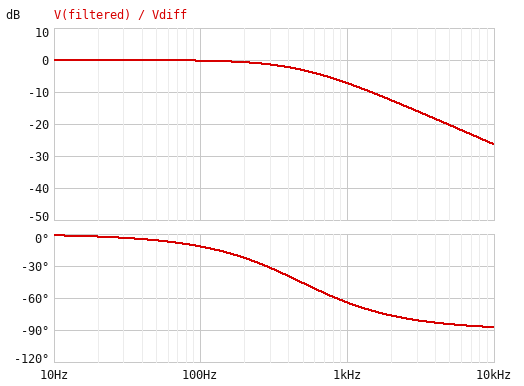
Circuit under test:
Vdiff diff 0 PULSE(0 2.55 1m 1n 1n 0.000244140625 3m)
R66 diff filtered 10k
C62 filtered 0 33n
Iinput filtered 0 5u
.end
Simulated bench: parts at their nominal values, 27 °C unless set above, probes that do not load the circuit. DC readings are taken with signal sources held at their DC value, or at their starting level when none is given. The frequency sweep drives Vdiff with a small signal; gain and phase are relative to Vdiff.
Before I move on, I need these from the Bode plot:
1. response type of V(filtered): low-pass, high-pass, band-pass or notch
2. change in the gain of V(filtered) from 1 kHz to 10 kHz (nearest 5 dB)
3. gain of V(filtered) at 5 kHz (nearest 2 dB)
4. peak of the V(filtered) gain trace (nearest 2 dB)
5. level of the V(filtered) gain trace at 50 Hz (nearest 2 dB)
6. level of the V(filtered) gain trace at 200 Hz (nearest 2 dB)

low-pass
-20 dB
-20 dB
0 dB
0 dB
0 dB
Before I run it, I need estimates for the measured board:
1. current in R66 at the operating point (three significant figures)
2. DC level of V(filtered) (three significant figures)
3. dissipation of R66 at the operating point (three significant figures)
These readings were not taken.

5.00 µA
-50.0 mV
250 nW
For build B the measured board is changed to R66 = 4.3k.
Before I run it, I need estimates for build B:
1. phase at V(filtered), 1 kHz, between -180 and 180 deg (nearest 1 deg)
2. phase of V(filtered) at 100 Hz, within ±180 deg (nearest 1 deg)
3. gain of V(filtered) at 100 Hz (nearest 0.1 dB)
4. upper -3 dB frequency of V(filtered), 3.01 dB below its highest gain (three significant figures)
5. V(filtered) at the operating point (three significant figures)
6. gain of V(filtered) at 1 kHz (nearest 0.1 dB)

-42 deg
-5 deg
0 dB
1.12 kHz
-21.5 mV
-2.5 dB
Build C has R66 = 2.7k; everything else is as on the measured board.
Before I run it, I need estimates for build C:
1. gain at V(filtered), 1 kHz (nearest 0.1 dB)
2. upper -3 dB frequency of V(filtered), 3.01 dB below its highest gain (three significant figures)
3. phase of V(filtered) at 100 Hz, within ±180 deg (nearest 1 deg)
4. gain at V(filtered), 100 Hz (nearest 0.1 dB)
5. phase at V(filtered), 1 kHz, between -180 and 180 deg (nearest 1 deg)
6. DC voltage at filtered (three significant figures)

-1.2 dB
1.79 kHz
-3 deg
0 dB
-29 deg
-13.5 mV
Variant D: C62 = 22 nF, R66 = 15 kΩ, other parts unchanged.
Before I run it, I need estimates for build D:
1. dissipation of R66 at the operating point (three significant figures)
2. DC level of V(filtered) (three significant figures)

375 nW
-75.0 mV
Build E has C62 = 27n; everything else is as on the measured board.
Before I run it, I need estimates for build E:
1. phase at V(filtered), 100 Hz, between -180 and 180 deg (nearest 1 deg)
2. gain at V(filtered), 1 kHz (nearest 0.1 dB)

-10 deg
-5.9 dB
